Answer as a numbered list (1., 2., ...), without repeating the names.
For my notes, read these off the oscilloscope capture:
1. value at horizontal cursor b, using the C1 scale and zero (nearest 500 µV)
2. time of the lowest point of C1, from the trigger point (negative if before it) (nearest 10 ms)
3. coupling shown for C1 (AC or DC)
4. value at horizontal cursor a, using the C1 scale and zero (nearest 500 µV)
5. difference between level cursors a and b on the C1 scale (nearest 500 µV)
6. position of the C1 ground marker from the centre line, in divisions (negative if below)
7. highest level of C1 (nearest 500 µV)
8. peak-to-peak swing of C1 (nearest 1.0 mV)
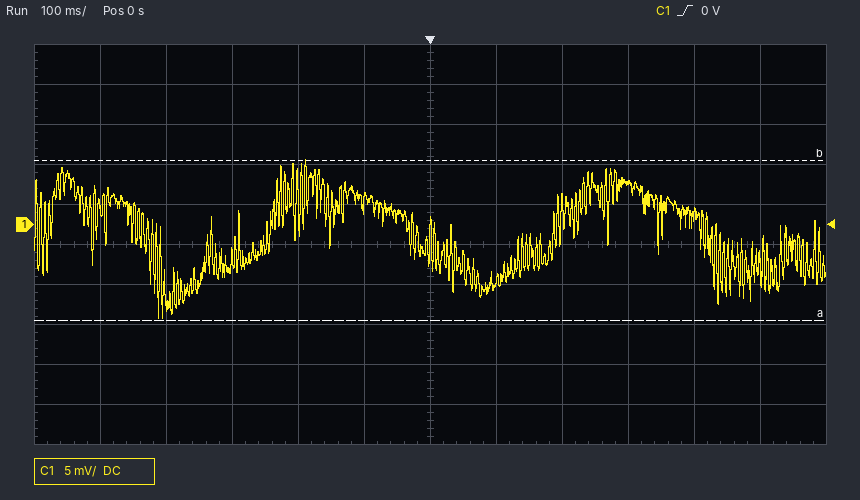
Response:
1. 8.0 mV
2. -410 ms
3. DC
4. -12.0 mV
5. 20.0 mV
6. +0.5 div
7. 8.0 mV
8. 20.0 mV
